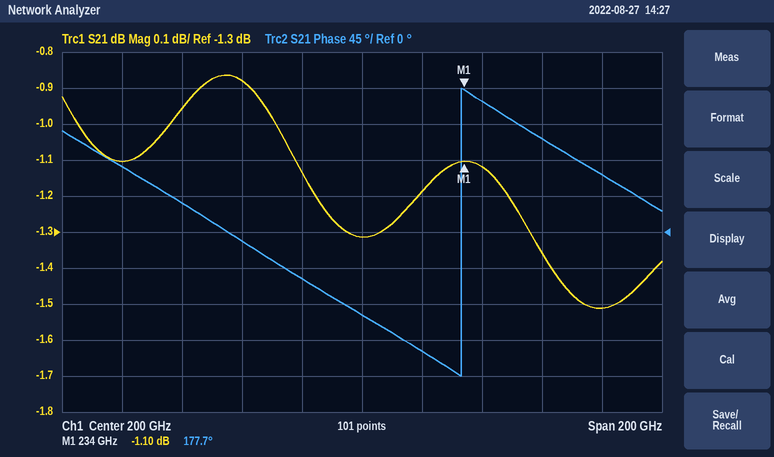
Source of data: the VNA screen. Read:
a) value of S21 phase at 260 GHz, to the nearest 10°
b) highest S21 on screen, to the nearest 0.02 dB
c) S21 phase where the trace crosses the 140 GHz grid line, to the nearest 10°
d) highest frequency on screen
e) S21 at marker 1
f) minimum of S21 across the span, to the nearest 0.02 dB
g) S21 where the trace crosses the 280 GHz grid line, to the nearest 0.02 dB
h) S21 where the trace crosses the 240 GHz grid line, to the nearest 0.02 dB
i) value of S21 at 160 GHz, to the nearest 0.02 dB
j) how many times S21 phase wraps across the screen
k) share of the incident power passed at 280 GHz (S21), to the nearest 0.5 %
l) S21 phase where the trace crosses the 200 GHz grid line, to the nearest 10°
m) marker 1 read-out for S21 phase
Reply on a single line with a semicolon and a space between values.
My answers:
120°; -0.86 dB; 40°; 300 GHz; -1.10 dB; -1.52 dB; -1.52 dB; -1.12 dB; -0.88 dB; 1; 70.5 %; -100°; 177.7°
